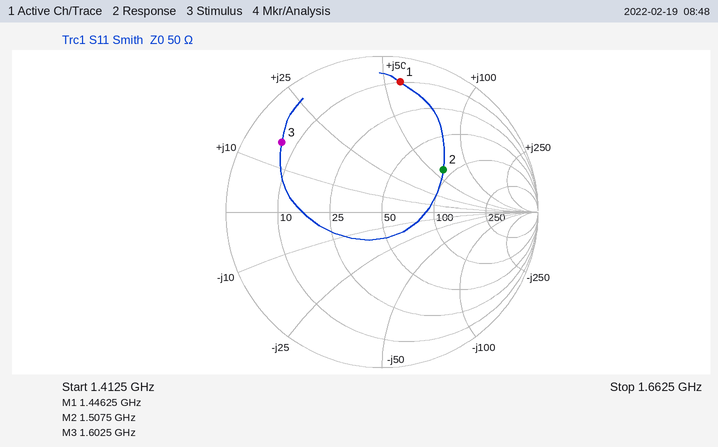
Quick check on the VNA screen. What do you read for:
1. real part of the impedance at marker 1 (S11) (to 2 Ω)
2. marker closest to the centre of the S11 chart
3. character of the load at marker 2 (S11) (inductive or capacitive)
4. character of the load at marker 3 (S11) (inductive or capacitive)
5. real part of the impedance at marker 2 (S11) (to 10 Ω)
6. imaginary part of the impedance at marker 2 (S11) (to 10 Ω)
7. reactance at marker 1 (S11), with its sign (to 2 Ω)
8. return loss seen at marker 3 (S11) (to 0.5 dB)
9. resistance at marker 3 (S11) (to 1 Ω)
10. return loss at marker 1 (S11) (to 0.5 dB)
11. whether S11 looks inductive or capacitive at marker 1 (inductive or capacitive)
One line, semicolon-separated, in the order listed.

10 Ω; marker 2; inductive; inductive; 90 Ω; +60 Ω; +56 Ω; 2.0 dB; 7 Ω; 1.5 dB; inductive
